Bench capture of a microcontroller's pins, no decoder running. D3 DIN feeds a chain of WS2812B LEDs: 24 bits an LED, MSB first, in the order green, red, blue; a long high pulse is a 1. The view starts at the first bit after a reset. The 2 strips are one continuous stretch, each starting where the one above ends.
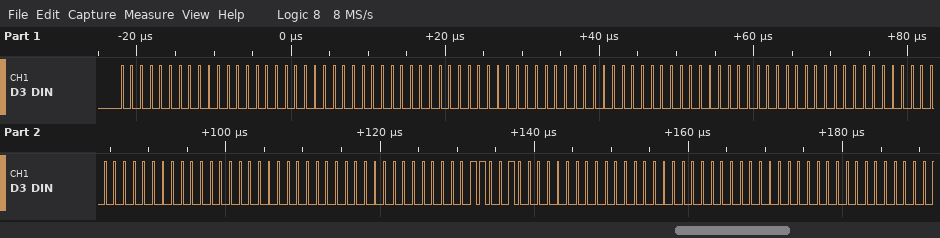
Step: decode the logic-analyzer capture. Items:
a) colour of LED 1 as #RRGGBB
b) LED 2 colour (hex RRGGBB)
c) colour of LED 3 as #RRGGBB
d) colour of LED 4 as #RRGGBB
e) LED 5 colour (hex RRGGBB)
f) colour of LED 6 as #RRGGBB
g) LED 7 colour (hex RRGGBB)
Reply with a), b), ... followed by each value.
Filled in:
a) #000000
b) #000000
c) #000000
d) #000000
e) #000000
f) #001900
g) #000000
